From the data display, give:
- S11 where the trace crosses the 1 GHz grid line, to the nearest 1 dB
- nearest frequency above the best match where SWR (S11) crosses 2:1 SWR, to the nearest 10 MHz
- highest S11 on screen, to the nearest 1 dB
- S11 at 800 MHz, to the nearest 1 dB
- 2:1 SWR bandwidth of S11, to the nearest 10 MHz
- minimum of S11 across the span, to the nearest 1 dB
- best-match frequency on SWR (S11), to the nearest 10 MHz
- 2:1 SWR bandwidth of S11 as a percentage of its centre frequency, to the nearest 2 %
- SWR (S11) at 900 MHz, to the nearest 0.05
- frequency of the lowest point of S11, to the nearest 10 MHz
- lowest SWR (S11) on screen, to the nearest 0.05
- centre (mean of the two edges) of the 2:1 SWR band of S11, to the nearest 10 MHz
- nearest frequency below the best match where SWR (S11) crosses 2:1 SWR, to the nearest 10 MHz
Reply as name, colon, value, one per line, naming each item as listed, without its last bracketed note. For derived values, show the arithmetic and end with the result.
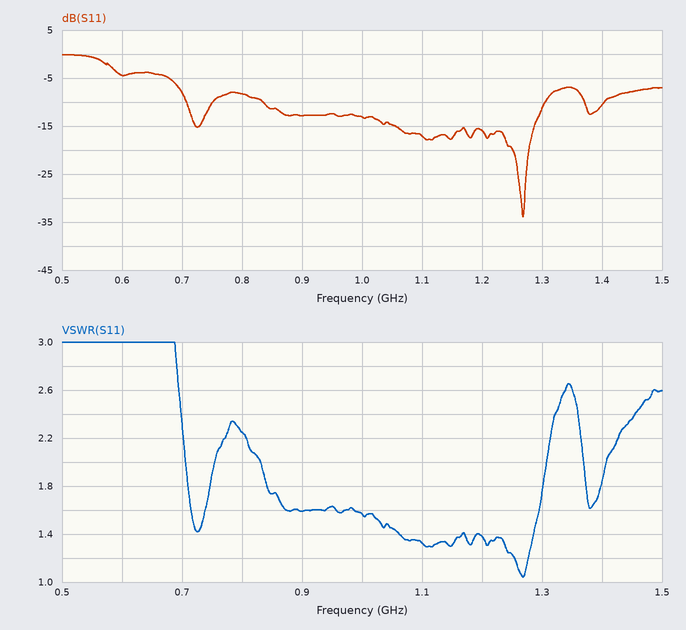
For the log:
S11 where the trace crosses the 1 GHz grid line, to the nearest 1 dB: -13 dB
nearest frequency above the best match where SWR (S11) crosses 2:1 SWR, to the nearest 10 MHz: 1.31 GHz
highest S11 on screen, to the nearest 1 dB: 0 dB
S11 at 800 MHz, to the nearest 1 dB: -8 dB
2:1 SWR bandwidth of S11, to the nearest 10 MHz: 1.31 GHz − 830 MHz = 480 MHz
minimum of S11 across the span, to the nearest 1 dB: -34 dB
best-match frequency on SWR (S11), to the nearest 10 MHz: 1.27 GHz
2:1 SWR bandwidth of S11 as a percentage of its centre frequency, to the nearest 2 %: 480 MHz / 1.07 GHz ≈ 44.9 %, so 44 % to the nearest 2 %
SWR (S11) at 900 MHz, to the nearest 0.05: 1.60
frequency of the lowest point of S11, to the nearest 10 MHz: 1.27 GHz
lowest SWR (S11) on screen, to the nearest 0.05: 1.05
centre (mean of the two edges) of the 2:1 SWR band of S11, to the nearest 10 MHz: 1.07 GHz
nearest frequency below the best match where SWR (S11) crosses 2:1 SWR, to the nearest 10 MHz: 830 MHz
